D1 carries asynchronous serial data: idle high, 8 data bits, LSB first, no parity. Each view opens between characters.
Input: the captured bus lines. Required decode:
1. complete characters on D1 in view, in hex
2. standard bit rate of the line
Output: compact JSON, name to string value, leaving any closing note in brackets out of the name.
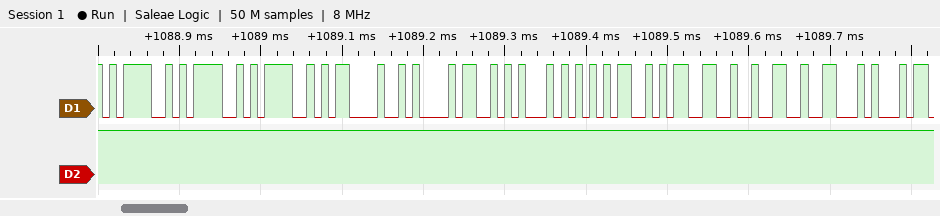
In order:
{"complete characters on D1 in view, in hex": "3D, 3D, 3D, 0D, 0A, 53, 54, 4D, 33, 32, 46", "standard bit rate of the line": "115200 baud"}
